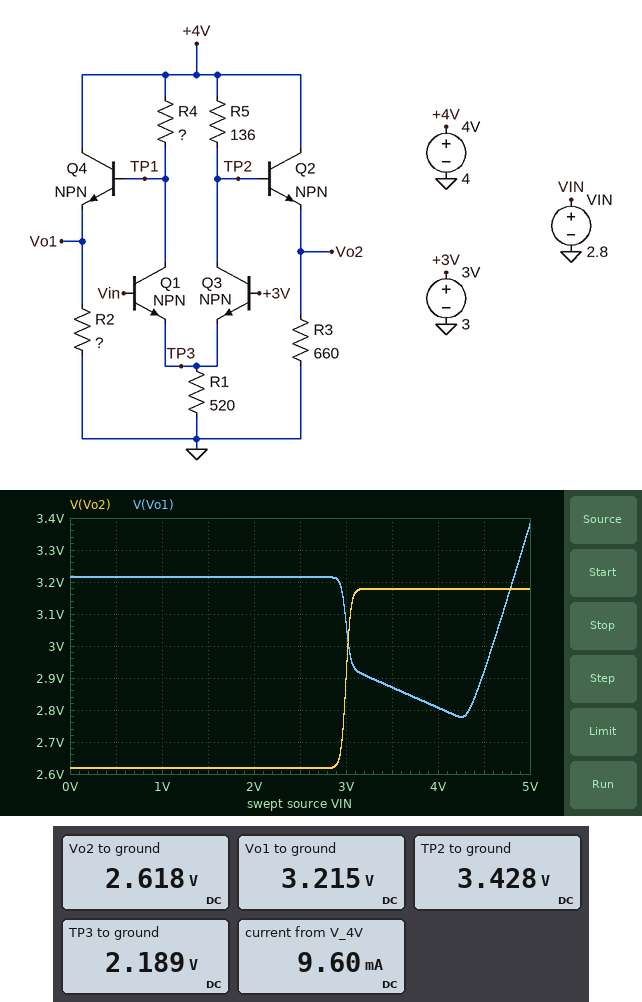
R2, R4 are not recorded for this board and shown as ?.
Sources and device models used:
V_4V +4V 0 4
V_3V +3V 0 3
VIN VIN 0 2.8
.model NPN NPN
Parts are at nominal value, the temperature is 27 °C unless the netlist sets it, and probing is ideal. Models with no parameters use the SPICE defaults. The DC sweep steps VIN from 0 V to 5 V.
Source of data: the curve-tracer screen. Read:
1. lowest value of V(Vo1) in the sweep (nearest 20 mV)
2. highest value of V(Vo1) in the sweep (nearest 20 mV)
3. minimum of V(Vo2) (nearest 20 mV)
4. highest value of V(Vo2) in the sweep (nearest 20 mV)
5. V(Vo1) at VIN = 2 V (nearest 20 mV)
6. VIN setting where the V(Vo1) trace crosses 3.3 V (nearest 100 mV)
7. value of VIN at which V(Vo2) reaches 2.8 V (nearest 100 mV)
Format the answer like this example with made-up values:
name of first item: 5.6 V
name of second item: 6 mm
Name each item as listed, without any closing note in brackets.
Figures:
lowest value of V(Vo1) in the sweep: 2.78 V
highest value of V(Vo1) in the sweep: 3.38 V
minimum of V(Vo2): 2.62 V
highest value of V(Vo2) in the sweep: 3.18 V
V(Vo1) at VIN = 2 V: 3.22 V
VIN setting where the V(Vo1) trace crosses 3.3 V: 4.9 V
value of VIN at which V(Vo2) reaches 2.8 V: 3.0 V
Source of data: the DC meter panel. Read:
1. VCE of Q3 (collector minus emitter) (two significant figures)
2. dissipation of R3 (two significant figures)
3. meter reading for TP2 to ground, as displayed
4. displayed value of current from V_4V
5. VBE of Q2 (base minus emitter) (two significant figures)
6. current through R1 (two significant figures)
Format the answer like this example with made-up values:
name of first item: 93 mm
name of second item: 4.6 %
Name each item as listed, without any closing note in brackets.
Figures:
VCE of Q3 (collector minus emitter): 1.2 V
dissipation of R3: 10 mW
meter reading for TP2 to ground, as displayed: 3.428 V
displayed value of current from V_4V: 9.60 mA
VBE of Q2 (base minus emitter): 810 mV
current through R1: 4.2 mA
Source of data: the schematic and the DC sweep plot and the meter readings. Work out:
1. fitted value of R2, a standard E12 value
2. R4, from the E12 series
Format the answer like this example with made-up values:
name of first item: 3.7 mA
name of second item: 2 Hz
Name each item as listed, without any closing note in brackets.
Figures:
fitted value of R2, a standard E12 value: 2.2 kΩ
R4, from the E12 series: 68 Ω
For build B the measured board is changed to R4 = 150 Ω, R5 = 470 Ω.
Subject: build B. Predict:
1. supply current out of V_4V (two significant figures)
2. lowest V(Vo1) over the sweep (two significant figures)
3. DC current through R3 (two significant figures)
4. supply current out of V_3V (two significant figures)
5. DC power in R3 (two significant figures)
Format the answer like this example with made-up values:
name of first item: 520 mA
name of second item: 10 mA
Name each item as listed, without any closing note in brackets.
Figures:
supply current out of V_4V: 7.4 mA
lowest V(Vo1) over the sweep: 2.4 V
DC current through R3: 2.2 mA
supply current out of V_3V: 490 µA
DC power in R3: 3.2 mW
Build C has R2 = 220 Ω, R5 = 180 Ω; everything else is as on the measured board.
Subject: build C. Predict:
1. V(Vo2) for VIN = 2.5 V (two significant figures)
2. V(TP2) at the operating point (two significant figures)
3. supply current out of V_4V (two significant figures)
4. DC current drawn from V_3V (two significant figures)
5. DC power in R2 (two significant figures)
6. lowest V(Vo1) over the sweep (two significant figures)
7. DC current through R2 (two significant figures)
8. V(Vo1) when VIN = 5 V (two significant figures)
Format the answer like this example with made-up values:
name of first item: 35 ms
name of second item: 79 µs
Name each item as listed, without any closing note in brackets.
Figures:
V(Vo2) for VIN = 2.5 V: 2.4 V
V(TP2) at the operating point: 3.2 V
supply current out of V_4V: 22 mA
DC current drawn from V_3V: 42 µA
DC power in R2: 45 mW
lowest V(Vo1) over the sweep: 2.7 V
DC current through R2: 14 mA
V(Vo1) when VIN = 5 V: 3.3 V
